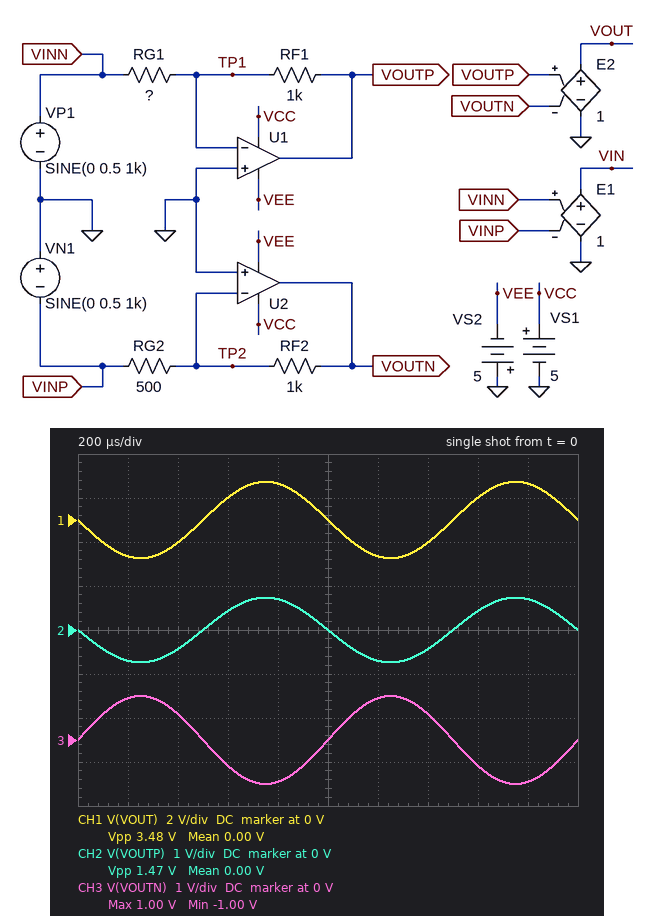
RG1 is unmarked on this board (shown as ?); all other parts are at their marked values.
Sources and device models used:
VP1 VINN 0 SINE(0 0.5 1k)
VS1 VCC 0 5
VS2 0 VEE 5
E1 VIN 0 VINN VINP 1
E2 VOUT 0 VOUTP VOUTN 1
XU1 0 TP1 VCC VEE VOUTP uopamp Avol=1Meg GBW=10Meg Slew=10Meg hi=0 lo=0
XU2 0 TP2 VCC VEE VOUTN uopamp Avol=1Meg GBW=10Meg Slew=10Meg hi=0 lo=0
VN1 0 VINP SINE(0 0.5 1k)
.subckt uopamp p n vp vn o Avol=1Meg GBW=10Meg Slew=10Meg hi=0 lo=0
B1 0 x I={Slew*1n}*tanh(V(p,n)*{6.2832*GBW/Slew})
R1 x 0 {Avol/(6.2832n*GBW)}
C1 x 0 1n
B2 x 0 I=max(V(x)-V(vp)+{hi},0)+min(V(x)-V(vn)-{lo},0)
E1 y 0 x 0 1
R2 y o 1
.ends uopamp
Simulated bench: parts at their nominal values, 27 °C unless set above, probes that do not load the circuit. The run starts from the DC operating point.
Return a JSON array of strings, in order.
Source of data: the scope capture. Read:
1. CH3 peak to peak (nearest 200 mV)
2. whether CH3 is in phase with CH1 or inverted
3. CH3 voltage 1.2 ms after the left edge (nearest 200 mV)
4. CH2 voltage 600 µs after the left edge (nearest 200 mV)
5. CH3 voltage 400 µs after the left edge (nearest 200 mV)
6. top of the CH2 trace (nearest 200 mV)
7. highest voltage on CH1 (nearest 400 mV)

["2.0 V", "inverted", "1.0 V", "400 mV", "600 mV", "800 mV", "1.6 V"]
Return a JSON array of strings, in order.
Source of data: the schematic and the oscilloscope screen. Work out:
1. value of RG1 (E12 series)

["680 Ω"]
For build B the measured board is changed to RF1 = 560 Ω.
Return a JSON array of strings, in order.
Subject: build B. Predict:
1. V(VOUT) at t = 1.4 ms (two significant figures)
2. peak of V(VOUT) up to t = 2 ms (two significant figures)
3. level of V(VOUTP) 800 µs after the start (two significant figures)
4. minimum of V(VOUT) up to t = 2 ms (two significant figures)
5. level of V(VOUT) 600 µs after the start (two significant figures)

["-830 mV", "1.4 V", "390 mV", "-1.4 V", "830 mV"]
